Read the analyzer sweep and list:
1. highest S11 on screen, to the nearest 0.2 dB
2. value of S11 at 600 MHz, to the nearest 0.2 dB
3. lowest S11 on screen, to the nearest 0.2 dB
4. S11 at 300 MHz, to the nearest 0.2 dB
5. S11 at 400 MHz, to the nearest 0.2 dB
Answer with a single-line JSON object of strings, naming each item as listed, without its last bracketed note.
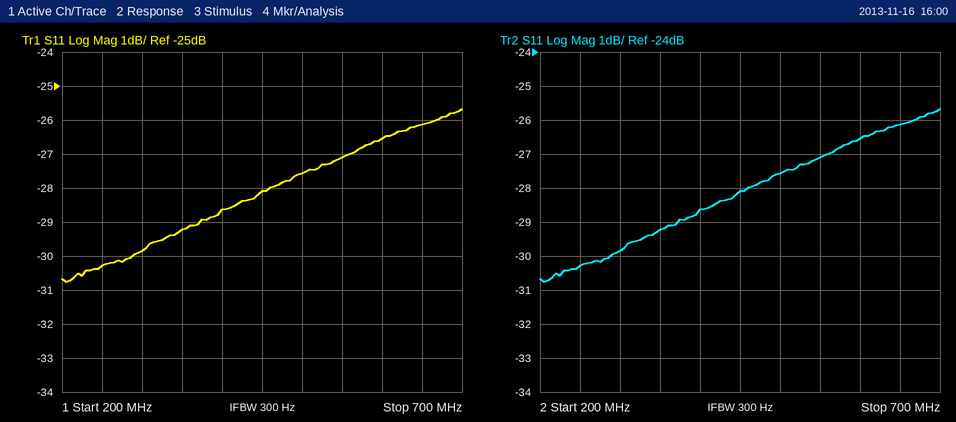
{"highest S11 on screen, to the nearest 0.2 dB": "-25.6 dB", "value of S11 at 600 MHz, to the nearest 0.2 dB": "-26.6 dB", "lowest S11 on screen, to the nearest 0.2 dB": "-30.8 dB", "S11 at 300 MHz, to the nearest 0.2 dB": "-29.8 dB", "S11 at 400 MHz, to the nearest 0.2 dB": "-28.6 dB"}
